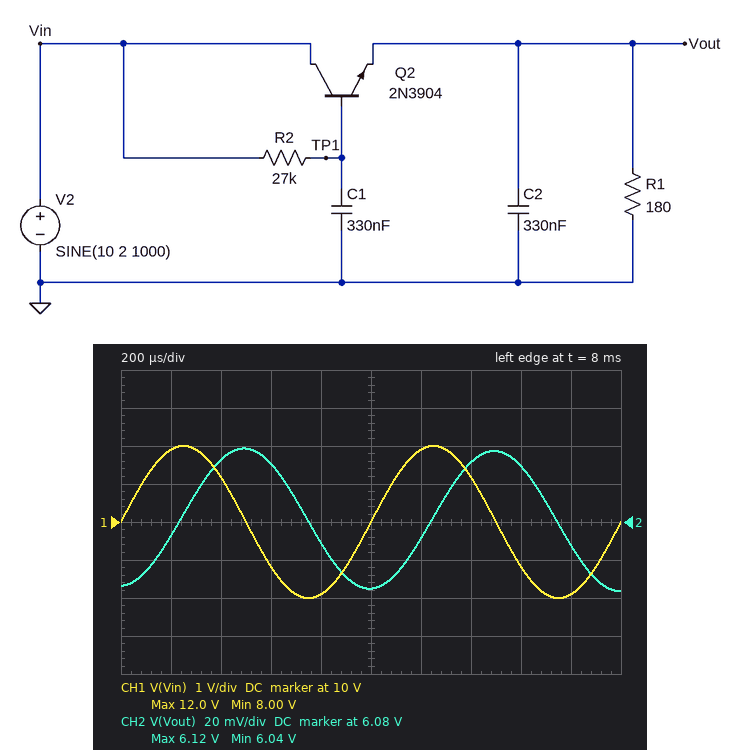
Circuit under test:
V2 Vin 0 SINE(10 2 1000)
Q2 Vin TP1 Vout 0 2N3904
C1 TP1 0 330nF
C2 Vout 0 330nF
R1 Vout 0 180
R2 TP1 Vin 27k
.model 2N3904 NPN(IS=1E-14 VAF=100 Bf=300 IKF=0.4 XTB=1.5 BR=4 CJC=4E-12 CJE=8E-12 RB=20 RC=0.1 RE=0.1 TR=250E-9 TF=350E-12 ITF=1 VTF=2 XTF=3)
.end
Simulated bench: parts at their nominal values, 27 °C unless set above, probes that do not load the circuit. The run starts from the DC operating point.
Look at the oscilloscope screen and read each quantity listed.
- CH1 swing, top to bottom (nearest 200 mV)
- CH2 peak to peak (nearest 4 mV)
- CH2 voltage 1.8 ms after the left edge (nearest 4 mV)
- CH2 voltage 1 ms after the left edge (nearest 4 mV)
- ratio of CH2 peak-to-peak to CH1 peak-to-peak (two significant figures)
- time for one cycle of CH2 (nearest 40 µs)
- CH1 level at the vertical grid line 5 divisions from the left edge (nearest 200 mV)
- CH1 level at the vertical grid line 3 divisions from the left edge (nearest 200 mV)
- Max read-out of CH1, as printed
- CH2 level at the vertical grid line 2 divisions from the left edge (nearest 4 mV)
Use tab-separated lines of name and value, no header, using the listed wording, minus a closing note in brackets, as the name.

CH1 swing, top to bottom	4.0 V
CH2 peak to peak	76 mV
CH2 voltage 1.8 ms after the left edge	6.068 V
CH2 voltage 1 ms after the left edge	6.044 V
ratio of CH2 peak-to-peak to CH1 peak-to-peak	0.019
time for one cycle of CH2	1.00 ms
CH1 level at the vertical grid line 5 divisions from the left edge	10.0 V
CH1 level at the vertical grid line 3 divisions from the left edge	8.8 V
Max read-out of CH1, as printed	12.0 V
CH2 level at the vertical grid line 2 divisions from the left edge	6.112 V
